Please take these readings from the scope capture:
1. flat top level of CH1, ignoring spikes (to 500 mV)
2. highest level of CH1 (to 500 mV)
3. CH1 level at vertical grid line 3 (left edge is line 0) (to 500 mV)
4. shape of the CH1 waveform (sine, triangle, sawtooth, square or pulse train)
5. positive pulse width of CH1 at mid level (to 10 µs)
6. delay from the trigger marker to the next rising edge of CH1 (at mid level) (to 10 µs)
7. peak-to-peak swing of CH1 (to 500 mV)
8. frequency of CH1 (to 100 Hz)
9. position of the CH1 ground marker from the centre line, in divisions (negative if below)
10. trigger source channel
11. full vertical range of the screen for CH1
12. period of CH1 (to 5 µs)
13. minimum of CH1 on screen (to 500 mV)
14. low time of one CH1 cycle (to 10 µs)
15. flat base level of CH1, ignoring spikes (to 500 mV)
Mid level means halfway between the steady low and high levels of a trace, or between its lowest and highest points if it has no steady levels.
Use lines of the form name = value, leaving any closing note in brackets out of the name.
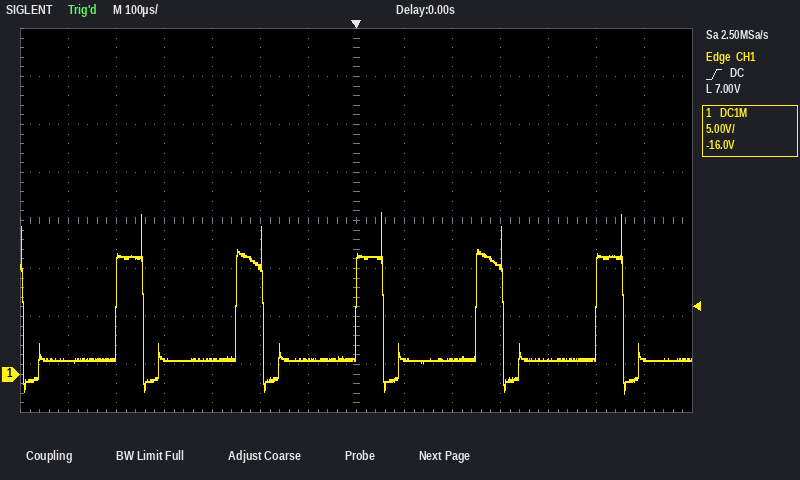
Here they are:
flat top level of CH1, ignoring spikes = 12.0 V
highest level of CH1 = 17.0 V
CH1 level at vertical grid line 3 (left edge is line 0) = 1.5 V
shape of the CH1 waveform = pulse train
positive pulse width of CH1 at mid level = 60 µs
delay from the trigger marker to the next rising edge of CH1 (at mid level) = 250 µs
peak-to-peak swing of CH1 = 19.0 V
frequency of CH1 = 4.0 kHz
position of the CH1 ground marker from the centre line, in divisions = -3.2 div
trigger source channel = CH1
full vertical range of the screen for CH1 = 40 V
period of CH1 = 250 µs
minimum of CH1 on screen = -2.0 V
low time of one CH1 cycle = 190 µs
flat base level of CH1, ignoring spikes = 1.5 V
